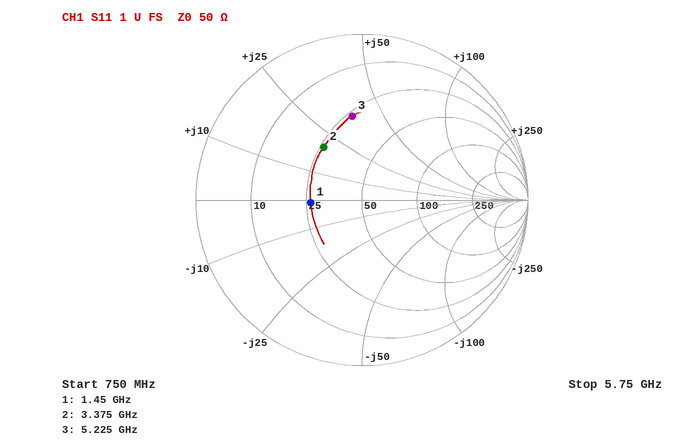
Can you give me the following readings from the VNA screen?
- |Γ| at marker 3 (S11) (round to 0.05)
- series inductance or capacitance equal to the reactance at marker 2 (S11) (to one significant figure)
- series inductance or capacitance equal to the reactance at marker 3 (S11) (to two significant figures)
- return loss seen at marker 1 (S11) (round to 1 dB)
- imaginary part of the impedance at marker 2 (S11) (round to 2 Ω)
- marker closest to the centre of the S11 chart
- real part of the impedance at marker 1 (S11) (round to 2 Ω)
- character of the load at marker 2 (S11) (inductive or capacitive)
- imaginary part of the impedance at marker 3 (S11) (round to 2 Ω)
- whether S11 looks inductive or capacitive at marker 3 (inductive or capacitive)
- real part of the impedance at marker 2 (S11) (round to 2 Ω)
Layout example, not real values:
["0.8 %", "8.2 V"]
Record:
["0.50", "900 pH", "1.1 nH", "10 dB", "+20 Ω", "marker 1", "26 Ω", "inductive", "+36 Ω", "inductive", "26 Ω"]
